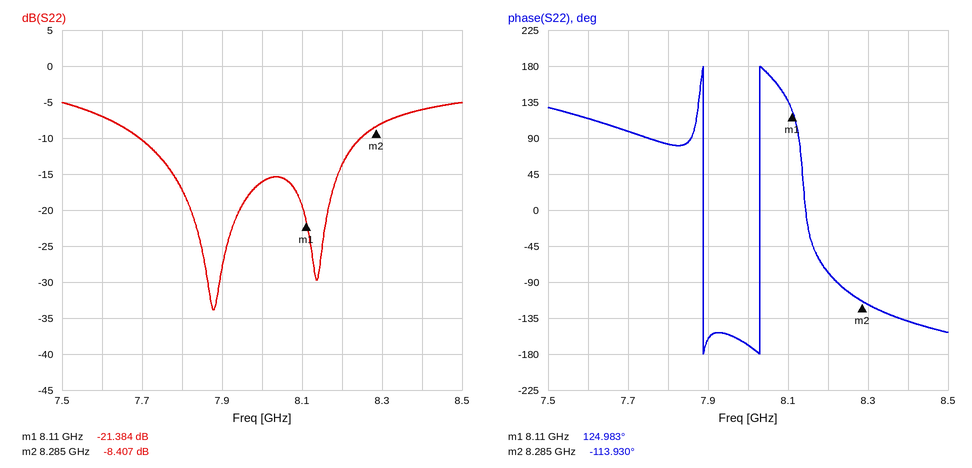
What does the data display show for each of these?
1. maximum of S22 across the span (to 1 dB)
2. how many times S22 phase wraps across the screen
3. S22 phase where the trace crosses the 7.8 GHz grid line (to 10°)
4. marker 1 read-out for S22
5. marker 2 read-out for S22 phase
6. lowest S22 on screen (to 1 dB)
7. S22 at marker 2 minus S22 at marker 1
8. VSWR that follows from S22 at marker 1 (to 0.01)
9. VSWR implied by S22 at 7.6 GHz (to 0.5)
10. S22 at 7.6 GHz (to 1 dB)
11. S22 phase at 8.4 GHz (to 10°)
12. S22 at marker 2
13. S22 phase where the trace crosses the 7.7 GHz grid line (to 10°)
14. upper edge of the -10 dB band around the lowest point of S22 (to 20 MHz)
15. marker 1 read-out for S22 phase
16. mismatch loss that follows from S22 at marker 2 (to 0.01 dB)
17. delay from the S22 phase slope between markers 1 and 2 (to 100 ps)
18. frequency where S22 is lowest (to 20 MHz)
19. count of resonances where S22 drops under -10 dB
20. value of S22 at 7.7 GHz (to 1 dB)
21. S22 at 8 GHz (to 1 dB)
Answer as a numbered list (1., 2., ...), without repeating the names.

1. -5 dB
2. 2
3. 80°
4. -21.384 dB
5. -113.930°
6. -34 dB
7. 12.977 dB
8. 1.19
9. 2.5
10. -7 dB
11. -140°
12. -8.407 dB
13. 100°
14. 8.24 GHz
15. 124.983°
16. 0.68 dB
17. 3.8 ns
18. 7.88 GHz
19. 2
20. -10 dB
21. -16 dB
